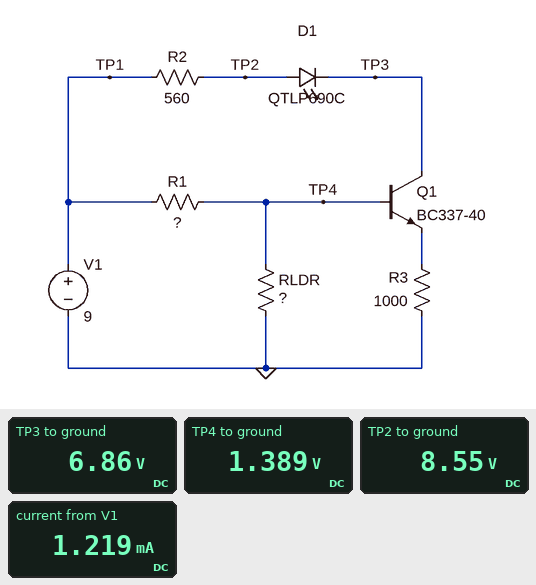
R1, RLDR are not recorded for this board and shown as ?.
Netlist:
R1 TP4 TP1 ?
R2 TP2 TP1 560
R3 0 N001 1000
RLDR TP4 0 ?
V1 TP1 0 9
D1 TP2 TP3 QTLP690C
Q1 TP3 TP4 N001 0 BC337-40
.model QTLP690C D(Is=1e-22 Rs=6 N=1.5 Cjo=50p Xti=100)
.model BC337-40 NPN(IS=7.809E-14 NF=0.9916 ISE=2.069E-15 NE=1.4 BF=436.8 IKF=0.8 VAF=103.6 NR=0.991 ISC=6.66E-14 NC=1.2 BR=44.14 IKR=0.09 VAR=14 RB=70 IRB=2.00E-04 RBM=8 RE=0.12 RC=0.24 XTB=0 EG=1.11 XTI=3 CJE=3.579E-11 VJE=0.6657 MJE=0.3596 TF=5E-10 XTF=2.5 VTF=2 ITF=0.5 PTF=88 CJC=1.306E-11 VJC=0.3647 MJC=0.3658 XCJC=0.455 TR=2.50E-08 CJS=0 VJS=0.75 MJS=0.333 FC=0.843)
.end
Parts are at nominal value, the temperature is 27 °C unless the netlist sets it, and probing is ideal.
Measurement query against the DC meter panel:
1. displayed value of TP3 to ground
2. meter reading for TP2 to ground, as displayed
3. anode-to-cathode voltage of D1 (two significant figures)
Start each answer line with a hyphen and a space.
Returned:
- 6.86 V
- 8.55 V
- 1.7 V
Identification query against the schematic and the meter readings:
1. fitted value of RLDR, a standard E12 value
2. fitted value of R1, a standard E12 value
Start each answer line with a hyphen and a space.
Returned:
- 3.3 kΩ
- 18 kΩ
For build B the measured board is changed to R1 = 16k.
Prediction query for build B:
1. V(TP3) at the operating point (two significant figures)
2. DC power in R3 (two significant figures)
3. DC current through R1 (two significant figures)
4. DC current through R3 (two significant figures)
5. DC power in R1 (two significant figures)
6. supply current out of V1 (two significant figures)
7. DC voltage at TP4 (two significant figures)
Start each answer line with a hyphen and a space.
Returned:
- 6.8 V
- 880 µW
- 470 µA
- 940 µA
- 3.5 mW
- 1.4 mA
- 1.5 V
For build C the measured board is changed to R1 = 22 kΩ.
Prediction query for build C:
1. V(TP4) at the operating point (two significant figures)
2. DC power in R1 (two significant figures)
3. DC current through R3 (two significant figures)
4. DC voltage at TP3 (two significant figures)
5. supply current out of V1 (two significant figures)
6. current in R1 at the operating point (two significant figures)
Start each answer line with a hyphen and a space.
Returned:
- 1.2 V
- 2.8 mW
- 590 µA
- 7.0 V
- 940 µA
- 360 µA
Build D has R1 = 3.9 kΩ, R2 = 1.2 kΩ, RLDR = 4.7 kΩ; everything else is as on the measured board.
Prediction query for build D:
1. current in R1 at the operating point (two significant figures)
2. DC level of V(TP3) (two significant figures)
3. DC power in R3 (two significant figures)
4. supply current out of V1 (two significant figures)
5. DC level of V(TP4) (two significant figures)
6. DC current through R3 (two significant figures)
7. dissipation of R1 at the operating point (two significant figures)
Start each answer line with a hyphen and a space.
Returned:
- 1.2 mA
- 3.5 V
- 12 mW
- 4.4 mA
- 4.2 V
- 3.5 mA
- 6.0 mW
